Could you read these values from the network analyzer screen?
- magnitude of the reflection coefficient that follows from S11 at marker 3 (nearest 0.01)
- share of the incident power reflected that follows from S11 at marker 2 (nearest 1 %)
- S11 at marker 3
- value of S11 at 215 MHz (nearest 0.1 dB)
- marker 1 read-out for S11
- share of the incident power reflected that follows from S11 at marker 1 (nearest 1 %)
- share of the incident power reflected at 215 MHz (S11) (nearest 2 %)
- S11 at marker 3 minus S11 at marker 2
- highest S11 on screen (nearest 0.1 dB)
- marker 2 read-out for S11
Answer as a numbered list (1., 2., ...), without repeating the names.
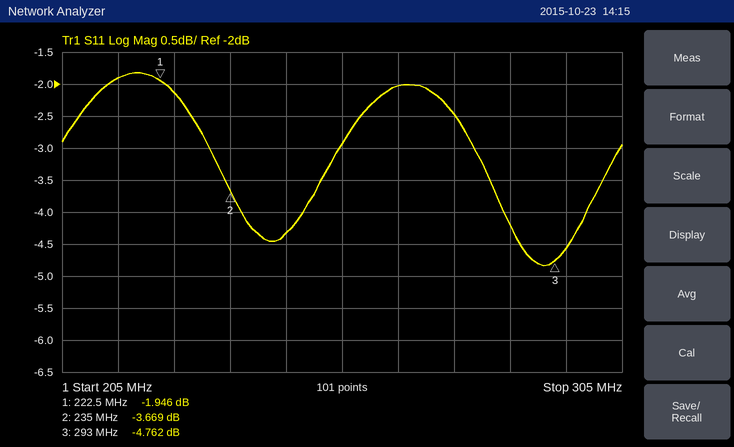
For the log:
1. 0.58
2. 43 %
3. -4.762 dB
4. -1.9 dB
5. -1.946 dB
6. 64 %
7. 64 %
8. -1.093 dB
9. -1.8 dB
10. -3.669 dB
